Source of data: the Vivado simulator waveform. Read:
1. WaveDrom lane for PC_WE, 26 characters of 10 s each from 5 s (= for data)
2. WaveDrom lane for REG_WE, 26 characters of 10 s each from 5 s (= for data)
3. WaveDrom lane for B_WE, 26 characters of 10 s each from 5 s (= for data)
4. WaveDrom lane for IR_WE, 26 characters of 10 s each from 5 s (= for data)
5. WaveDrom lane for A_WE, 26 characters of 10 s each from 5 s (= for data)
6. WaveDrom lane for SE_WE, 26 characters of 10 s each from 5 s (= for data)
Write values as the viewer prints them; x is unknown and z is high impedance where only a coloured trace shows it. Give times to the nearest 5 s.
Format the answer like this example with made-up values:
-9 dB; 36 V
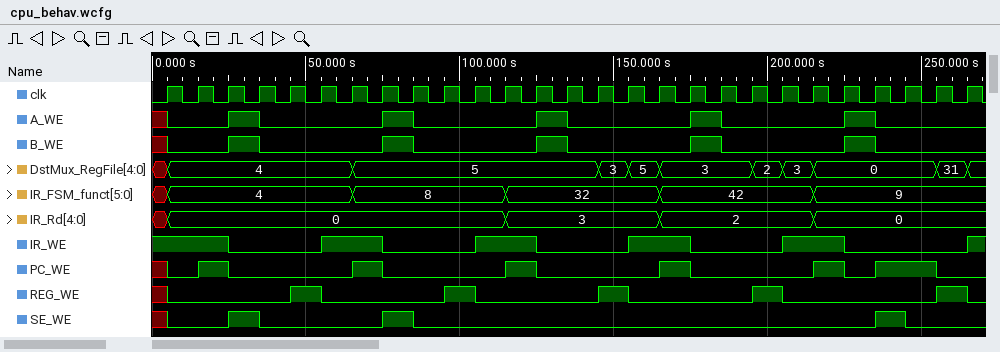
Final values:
{name: 'PC_WE', wave: '010...10...10...10...101.0'}; {name: 'REG_WE', wave: '0...10...10...10...10....1'}; {name: 'B_WE', wave: '0.10...10...10...10...10..'}; {name: 'IR_WE', wave: '1.0..1.0..1.0..1.0..1.0...'}; {name: 'A_WE', wave: '0.10...10...10...10...10..'}; {name: 'SE_WE', wave: '0.10...10..............10.'}
